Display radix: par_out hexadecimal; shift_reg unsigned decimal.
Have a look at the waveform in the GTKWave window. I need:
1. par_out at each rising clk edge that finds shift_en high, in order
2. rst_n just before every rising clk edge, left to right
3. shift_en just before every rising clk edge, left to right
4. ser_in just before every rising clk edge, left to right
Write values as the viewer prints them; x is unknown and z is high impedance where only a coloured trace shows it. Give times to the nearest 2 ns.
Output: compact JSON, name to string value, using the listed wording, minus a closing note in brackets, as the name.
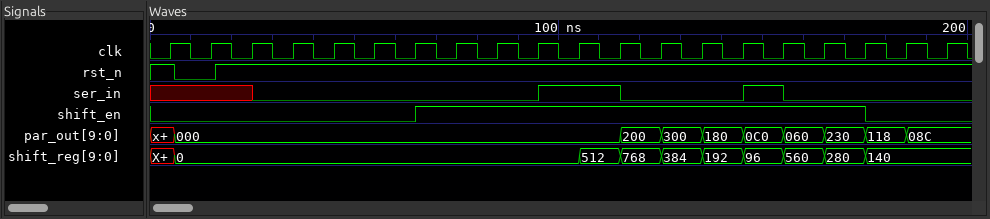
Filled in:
{"par_out at each rising clk edge that finds shift_en high, in order": "000, 000, 000, 000, 000, 200, 300, 180, 0C0, 060, 230", "rst_n just before every rising clk edge, left to right": "1 0 1 1 1 1 1 1 1 1 1 1 1 1 1 1 1 1 1 1", "shift_en just before every rising clk edge, left to right": "0 0 0 0 0 0 0 1 1 1 1 1 1 1 1 1 1 1 0 0", "ser_in just before every rising clk edge, left to right": "x x x 0 0 0 0 0 0 0 1 1 0 0 0 1 0 0 0 0"}
